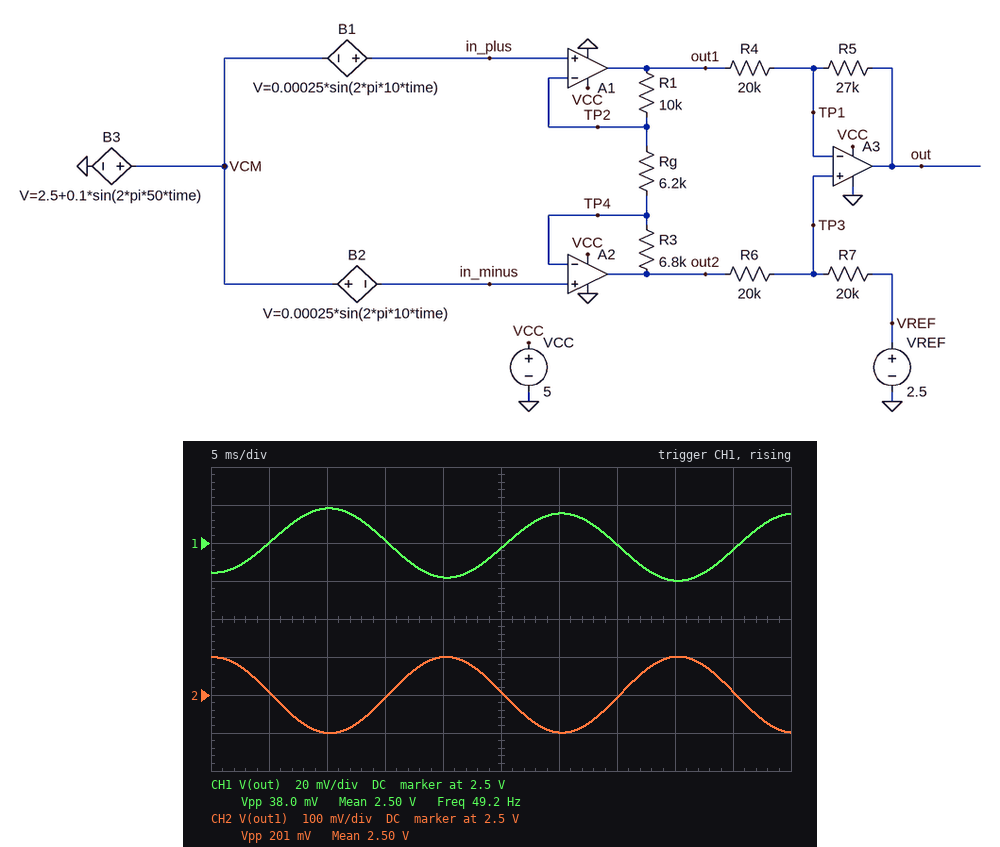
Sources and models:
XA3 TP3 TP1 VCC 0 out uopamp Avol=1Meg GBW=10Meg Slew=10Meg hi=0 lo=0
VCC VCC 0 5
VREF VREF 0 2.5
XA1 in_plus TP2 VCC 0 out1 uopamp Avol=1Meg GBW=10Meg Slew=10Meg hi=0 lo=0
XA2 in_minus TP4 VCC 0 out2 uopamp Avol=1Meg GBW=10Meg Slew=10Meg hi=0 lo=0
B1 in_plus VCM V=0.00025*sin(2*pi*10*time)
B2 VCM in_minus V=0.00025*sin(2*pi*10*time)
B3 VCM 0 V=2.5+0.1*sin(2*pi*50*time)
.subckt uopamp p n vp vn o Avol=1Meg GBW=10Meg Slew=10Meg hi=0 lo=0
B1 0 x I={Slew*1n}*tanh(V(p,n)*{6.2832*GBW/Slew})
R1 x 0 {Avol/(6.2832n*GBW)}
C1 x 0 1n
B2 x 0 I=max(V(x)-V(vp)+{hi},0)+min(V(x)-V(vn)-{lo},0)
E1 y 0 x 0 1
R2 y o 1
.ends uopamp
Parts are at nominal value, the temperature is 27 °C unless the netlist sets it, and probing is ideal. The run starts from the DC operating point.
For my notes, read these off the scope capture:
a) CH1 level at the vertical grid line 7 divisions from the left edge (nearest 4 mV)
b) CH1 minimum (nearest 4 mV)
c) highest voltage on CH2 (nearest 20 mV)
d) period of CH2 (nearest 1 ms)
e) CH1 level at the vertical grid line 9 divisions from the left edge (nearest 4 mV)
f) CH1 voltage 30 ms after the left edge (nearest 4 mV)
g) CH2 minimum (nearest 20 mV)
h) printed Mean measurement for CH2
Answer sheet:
2.500 V
2.480 V
2.60 V
20 ms
2.496 V
2.516 V
2.40 V
2.50 V
